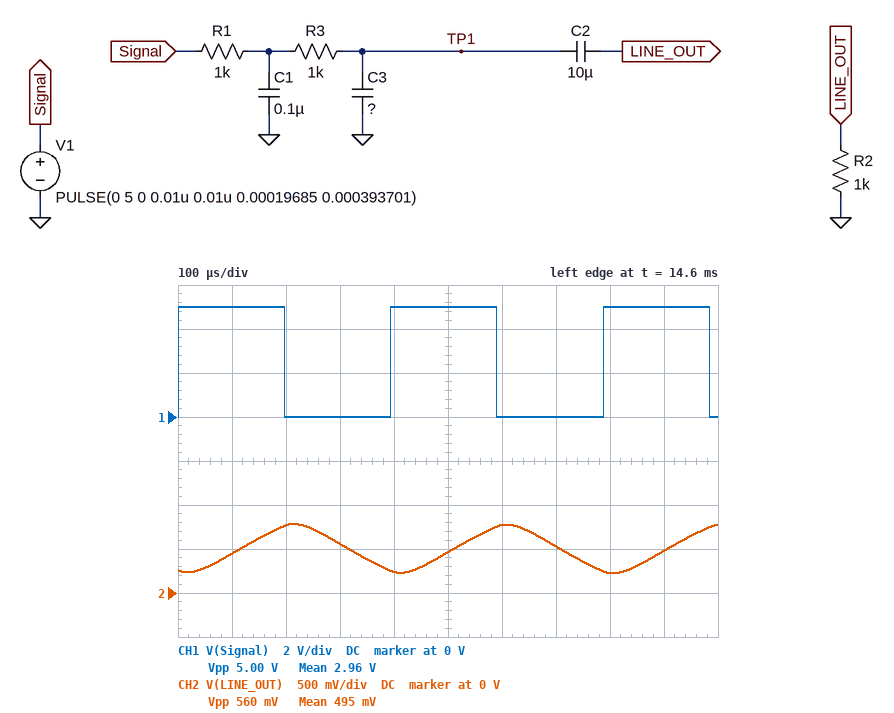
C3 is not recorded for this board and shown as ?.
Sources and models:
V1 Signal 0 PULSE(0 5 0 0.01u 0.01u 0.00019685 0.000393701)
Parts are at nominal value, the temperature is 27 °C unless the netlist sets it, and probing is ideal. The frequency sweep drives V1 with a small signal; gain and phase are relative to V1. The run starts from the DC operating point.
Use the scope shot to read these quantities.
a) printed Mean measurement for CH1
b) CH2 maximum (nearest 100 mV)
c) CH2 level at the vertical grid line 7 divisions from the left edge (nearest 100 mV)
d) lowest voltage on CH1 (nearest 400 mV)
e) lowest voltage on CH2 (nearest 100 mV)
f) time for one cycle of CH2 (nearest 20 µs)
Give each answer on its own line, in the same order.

2.96 V
800 mV
500 mV
0 V
200 mV
400 µs
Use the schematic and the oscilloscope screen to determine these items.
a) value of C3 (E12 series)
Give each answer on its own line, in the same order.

270 nF
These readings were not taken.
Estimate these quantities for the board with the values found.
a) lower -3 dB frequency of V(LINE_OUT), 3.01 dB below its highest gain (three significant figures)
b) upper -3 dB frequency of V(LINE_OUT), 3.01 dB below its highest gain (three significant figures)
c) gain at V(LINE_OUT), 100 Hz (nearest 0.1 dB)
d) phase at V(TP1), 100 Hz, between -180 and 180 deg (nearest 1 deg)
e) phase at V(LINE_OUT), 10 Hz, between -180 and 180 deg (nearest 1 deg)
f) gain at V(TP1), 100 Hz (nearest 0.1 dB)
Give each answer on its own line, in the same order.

5.17 Hz
772 Hz
-9.7 dB
-15 deg
27 deg
-9.6 dB
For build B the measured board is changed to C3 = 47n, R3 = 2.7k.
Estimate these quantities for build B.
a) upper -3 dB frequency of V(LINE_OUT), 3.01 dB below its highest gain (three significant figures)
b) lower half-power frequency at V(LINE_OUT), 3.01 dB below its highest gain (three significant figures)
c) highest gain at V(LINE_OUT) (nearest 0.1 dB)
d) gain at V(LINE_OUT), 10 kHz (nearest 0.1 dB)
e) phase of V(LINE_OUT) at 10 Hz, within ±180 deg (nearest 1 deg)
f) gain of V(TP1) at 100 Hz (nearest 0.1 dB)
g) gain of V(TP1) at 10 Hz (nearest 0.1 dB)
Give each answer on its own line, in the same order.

1.70 kHz
3.36 Hz
-13.5 dB
-35.1 dB
18 deg
-13.4 dB
-8.5 dB
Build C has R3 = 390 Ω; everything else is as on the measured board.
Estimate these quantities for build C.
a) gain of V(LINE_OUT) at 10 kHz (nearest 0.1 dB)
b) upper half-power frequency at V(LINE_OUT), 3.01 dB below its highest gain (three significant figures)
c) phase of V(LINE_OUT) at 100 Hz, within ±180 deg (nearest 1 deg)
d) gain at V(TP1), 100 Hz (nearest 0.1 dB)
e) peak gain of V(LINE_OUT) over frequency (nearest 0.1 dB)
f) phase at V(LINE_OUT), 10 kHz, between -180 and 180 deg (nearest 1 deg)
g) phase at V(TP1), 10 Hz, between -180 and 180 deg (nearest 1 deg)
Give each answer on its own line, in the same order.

-34.1 dB
838 Hz
-4 deg
-7.6 dB
-7.7 dB
-140 deg
-25 deg
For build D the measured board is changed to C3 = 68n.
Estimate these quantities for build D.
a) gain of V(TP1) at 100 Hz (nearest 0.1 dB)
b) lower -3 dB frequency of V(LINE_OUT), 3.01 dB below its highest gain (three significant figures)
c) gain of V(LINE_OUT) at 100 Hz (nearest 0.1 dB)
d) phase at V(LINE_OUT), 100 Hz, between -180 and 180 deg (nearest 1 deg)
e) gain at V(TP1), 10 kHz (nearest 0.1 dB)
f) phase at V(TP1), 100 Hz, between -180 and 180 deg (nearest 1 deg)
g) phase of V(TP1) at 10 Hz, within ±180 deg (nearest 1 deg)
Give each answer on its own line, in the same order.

-9.5 dB
5.25 Hz
-9.6 dB
-1 deg
-30.1 dB
-10 deg
-30 deg
